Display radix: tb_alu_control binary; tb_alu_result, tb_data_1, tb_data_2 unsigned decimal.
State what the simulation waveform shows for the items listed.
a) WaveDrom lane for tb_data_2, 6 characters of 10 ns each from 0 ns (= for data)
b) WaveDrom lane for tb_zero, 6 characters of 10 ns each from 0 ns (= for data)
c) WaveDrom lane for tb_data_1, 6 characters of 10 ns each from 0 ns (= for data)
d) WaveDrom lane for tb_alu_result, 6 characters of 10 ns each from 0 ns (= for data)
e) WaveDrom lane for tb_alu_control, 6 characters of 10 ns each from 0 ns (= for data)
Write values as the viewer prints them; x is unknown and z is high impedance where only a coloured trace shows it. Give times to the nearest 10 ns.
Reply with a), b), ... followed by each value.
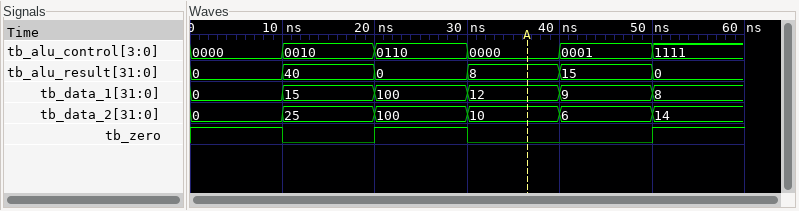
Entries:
a) {name: 'tb_data_2', wave: '======', data: '0 25 100 10 6 14'}
b) {name: 'tb_zero', wave: '1010.1'}
c) {name: 'tb_data_1', wave: '======', data: '0 15 100 12 9 8'}
d) {name: 'tb_alu_result', wave: '======', data: '0 40 0 8 15 0'}
e) {name: 'tb_alu_control', wave: '======', data: '0000 0010 0110 0000 0001 1111'}
